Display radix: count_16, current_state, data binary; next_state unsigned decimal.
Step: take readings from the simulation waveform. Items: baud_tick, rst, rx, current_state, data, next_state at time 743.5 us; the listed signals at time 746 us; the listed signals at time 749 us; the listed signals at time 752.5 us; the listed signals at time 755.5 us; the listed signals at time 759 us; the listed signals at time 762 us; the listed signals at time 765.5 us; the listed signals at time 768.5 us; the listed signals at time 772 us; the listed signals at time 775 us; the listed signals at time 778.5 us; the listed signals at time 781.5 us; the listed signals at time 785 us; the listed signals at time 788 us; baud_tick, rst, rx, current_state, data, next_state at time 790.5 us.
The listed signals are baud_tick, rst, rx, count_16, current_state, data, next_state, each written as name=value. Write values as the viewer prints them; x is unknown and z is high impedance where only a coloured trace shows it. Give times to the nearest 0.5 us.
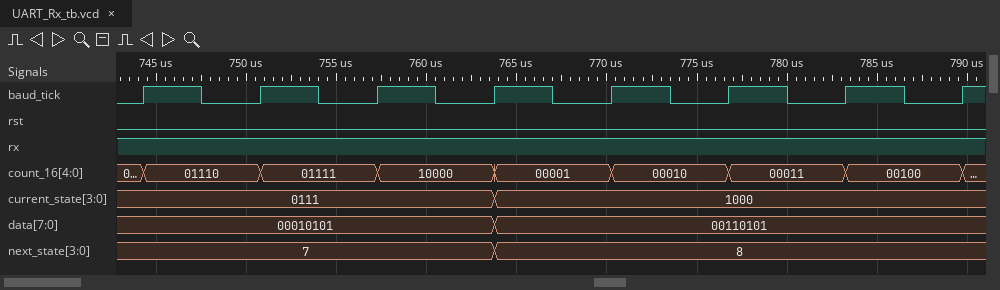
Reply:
baud_tick=0, rst=0, rx=1, current_state=0111, data=00010101, next_state=7
baud_tick=1, rst=0, rx=1, count_16=01110, current_state=0111, data=00010101, next_state=7
baud_tick=0, rst=0, rx=1, count_16=01110, current_state=0111, data=00010101, next_state=7
baud_tick=1, rst=0, rx=1, count_16=01111, current_state=0111, data=00010101, next_state=7
baud_tick=0, rst=0, rx=1, count_16=01111, current_state=0111, data=00010101, next_state=7
baud_tick=1, rst=0, rx=1, count_16=10000, current_state=0111, data=00010101, next_state=7
baud_tick=0, rst=0, rx=1, count_16=10000, current_state=0111, data=00010101, next_state=7
baud_tick=1, rst=0, rx=1, count_16=00001, current_state=1000, data=00110101, next_state=8
baud_tick=0, rst=0, rx=1, count_16=00001, current_state=1000, data=00110101, next_state=8
baud_tick=1, rst=0, rx=1, count_16=00010, current_state=1000, data=00110101, next_state=8
baud_tick=0, rst=0, rx=1, count_16=00010, current_state=1000, data=00110101, next_state=8
baud_tick=1, rst=0, rx=1, count_16=00011, current_state=1000, data=00110101, next_state=8
baud_tick=0, rst=0, rx=1, count_16=00011, current_state=1000, data=00110101, next_state=8
baud_tick=1, rst=0, rx=1, count_16=00100, current_state=1000, data=00110101, next_state=8
baud_tick=0, rst=0, rx=1, count_16=00100, current_state=1000, data=00110101, next_state=8
baud_tick=1, rst=0, rx=1, current_state=1000, data=00110101, next_state=8
